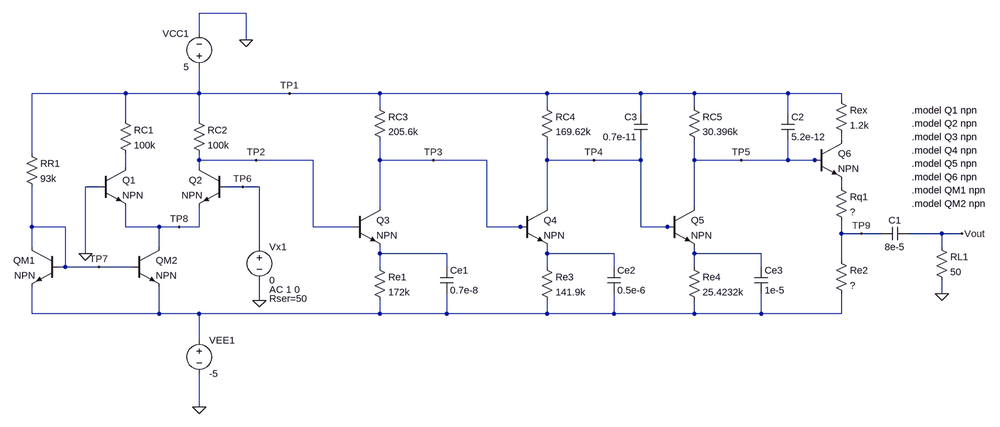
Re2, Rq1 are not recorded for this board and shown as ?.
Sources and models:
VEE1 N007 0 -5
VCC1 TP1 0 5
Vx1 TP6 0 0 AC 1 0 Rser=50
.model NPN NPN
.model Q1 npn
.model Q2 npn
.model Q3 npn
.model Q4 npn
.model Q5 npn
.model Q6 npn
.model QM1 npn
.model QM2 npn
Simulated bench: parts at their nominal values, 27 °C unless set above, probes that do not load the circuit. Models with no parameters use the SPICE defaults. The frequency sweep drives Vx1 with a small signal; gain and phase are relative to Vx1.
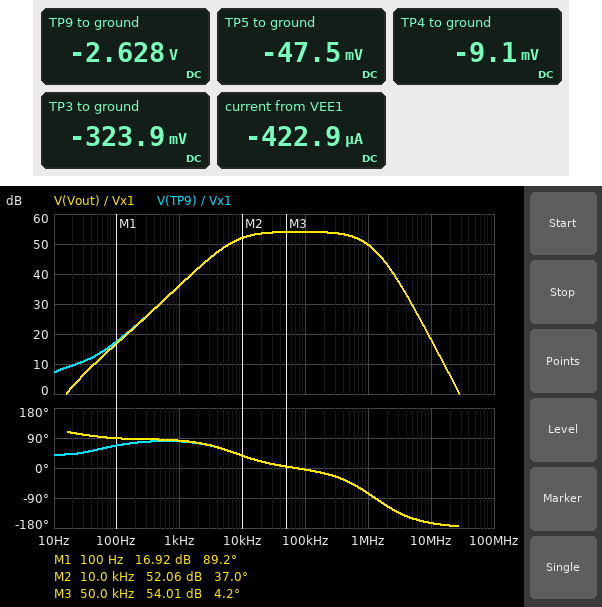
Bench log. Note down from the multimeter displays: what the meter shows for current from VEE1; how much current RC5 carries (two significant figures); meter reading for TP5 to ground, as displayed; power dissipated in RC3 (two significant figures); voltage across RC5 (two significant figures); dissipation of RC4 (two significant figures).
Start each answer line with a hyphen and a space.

- -422.9 µA
- 170 µA
- -47.5 mV
- 140 µW
- 5.0 V
- 150 µW
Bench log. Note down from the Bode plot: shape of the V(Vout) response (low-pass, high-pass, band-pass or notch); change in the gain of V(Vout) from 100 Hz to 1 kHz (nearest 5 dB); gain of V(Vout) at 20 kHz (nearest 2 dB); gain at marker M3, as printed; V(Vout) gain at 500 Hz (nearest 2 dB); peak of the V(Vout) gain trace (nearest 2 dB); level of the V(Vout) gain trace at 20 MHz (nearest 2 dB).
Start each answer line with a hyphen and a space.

- band-pass
- 20 dB
- 54 dB
- 54.01 dB
- 30 dB
- 54 dB
- 6 dB
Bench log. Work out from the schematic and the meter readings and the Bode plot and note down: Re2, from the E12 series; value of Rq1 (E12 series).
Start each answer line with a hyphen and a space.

- 680 kΩ
- 560 kΩ
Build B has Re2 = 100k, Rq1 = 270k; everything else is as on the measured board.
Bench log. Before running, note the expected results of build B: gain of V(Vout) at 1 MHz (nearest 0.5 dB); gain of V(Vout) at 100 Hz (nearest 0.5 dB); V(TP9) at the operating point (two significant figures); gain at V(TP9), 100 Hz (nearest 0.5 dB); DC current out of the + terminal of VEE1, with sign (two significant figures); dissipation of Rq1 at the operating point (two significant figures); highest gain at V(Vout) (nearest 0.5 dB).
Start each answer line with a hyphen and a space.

- 56.0 dB
- 23.5 dB
- -3.8 V
- 24.0 dB
- -430 µA
- 36 µW
- 60.5 dB
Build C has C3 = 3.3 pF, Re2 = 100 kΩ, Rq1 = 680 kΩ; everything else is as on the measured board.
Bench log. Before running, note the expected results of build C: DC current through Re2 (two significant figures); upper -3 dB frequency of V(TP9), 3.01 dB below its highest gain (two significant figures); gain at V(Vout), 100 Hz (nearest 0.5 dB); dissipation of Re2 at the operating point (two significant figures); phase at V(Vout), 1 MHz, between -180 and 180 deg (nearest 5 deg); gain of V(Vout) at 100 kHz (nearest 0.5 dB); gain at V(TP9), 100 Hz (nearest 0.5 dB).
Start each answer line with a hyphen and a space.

- 5.5 µA
- 950 kHz
- 15.5 dB
- 3.1 µW
- -60 deg
- 52.5 dB
- 16.0 dB
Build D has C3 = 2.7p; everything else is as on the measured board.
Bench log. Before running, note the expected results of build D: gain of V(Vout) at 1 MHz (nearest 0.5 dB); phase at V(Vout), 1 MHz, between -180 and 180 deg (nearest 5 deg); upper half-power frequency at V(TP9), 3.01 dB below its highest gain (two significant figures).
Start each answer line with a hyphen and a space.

- 51.0 dB
- -60 deg
- 970 kHz
